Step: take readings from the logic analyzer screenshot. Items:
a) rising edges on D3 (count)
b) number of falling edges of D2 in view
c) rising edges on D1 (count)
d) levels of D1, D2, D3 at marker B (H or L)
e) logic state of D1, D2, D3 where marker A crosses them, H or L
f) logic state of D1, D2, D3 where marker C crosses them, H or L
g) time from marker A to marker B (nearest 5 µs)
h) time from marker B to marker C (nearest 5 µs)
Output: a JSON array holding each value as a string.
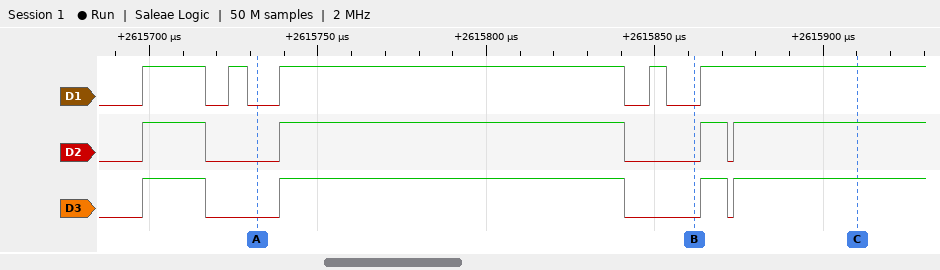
["4", "3", "5", "D1=L, D2=L, D3=L", "D1=L, D2=L, D3=L", "D1=H, D2=H, D3=H", "130 µs", "50 µs"]
